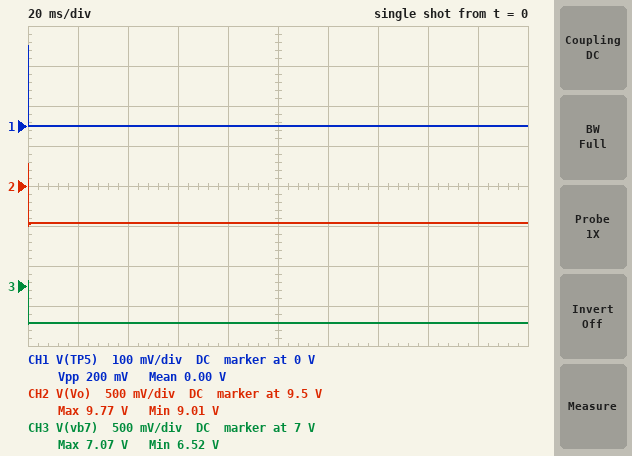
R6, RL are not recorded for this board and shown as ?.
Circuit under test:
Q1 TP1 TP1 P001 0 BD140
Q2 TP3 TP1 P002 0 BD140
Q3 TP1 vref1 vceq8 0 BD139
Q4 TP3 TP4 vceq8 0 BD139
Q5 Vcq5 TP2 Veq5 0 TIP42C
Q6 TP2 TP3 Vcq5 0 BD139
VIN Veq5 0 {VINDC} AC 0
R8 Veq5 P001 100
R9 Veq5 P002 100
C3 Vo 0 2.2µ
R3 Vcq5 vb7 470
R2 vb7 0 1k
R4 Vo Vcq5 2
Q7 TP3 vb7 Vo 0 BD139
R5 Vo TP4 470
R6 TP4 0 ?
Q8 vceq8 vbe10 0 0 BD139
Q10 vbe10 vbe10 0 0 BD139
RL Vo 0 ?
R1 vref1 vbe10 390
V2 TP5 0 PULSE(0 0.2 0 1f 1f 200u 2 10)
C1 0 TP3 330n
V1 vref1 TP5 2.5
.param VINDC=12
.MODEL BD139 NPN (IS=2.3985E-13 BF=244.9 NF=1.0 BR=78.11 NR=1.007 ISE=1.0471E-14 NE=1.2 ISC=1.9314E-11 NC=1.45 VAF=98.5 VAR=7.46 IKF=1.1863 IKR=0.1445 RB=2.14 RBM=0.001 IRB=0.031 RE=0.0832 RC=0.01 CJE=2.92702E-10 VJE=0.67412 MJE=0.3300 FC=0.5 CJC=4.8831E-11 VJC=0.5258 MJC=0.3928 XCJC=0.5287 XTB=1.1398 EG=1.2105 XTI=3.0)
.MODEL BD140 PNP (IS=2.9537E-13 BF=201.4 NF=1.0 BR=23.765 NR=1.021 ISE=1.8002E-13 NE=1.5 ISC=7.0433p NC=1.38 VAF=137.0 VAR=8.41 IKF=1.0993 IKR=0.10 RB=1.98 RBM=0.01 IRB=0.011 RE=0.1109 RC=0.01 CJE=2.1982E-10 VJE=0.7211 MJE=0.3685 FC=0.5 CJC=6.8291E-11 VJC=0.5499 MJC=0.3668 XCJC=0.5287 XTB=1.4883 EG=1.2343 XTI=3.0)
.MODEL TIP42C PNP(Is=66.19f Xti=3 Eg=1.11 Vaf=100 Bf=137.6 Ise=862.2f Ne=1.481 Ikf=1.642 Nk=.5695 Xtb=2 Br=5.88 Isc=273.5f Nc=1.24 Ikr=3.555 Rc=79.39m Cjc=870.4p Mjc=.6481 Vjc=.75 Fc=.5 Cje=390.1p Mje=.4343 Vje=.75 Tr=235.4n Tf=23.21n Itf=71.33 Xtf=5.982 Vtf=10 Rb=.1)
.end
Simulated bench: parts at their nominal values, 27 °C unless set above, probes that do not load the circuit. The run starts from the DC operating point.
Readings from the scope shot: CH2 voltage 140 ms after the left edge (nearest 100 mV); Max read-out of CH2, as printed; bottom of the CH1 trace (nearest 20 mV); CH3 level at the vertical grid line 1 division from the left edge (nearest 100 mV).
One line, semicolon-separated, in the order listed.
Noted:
9.0 V; 9.77 V; 0 V; 6.5 V
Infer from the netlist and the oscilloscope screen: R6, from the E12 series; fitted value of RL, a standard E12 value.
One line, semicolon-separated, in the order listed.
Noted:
180 Ω; 33 Ω
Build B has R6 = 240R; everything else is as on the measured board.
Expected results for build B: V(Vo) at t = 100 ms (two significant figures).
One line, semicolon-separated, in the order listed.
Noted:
7.4 V
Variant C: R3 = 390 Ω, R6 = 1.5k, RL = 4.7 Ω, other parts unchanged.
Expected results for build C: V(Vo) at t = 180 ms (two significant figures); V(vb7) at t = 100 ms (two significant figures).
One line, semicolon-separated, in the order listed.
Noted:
3.3 V; 3.4 V
